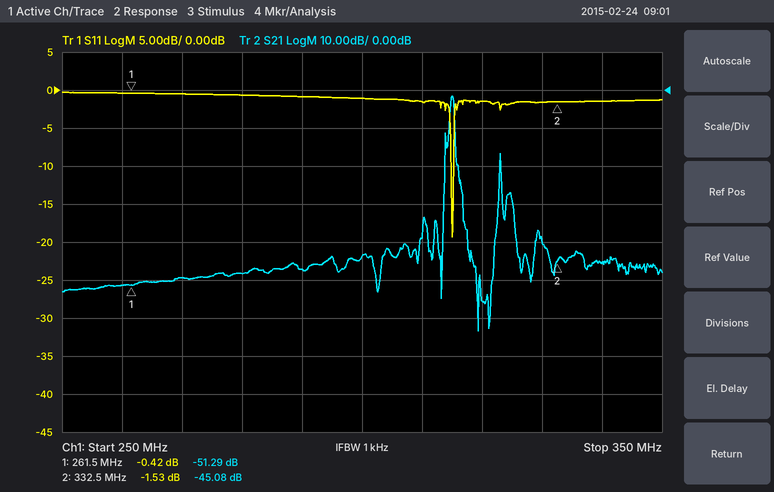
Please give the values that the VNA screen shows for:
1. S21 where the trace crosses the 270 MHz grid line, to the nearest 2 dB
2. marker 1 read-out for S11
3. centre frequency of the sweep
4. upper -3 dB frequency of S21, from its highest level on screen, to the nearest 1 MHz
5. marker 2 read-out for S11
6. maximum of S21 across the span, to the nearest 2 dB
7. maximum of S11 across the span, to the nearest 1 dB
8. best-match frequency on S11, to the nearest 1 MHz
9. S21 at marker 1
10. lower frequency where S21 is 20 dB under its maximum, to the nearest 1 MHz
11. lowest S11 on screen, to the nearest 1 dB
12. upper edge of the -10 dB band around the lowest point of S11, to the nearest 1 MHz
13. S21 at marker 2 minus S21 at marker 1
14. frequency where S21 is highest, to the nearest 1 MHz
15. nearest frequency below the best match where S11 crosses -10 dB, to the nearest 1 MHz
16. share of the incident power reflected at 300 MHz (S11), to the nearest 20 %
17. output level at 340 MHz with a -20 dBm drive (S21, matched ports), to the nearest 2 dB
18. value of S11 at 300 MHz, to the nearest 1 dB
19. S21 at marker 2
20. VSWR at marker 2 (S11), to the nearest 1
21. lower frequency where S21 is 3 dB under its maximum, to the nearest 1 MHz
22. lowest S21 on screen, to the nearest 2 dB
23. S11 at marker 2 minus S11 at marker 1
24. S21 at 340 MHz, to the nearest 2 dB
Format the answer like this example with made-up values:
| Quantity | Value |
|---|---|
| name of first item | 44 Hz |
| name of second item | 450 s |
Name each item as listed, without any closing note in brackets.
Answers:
| Quantity | Value |
|---|---|
| S21 where the trace crosses the 270 MHz grid line, to the nearest 2 dB | -50 dB |
| marker 1 read-out for S11 | -0.42 dB |
| centre frequency of the sweep | 300 MHz |
| upper -3 dB frequency of S21, from its highest level on screen, to the nearest 1 MHz | 315 MHz |
| marker 2 read-out for S11 | -1.53 dB |
| maximum of S21 across the span, to the nearest 2 dB | -2 dB |
| maximum of S11 across the span, to the nearest 1 dB | 0 dB |
| best-match frequency on S11, to the nearest 1 MHz | 315 MHz |
| S21 at marker 1 | -51.29 dB |
| lower frequency where S21 is 20 dB under its maximum, to the nearest 1 MHz | 314 MHz |
| lowest S11 on screen, to the nearest 1 dB | -19 dB |
| upper edge of the -10 dB band around the lowest point of S11, to the nearest 1 MHz | 315 MHz |
| S21 at marker 2 minus S21 at marker 1 | 6.21 dB |
| frequency where S21 is highest, to the nearest 1 MHz | 315 MHz |
| nearest frequency below the best match where S11 crosses -10 dB, to the nearest 1 MHz | 315 MHz |
| share of the incident power reflected at 300 MHz (S11), to the nearest 20 % | 80 % |
| output level at 340 MHz with a -20 dBm drive (S21, matched ports), to the nearest 2 dB | -66 dBm |
| value of S11 at 300 MHz, to the nearest 1 dB | -1 dB |
| S21 at marker 2 | -45.08 dB |
| VSWR at marker 2 (S11), to the nearest 1 | 11 |
| lower frequency where S21 is 3 dB under its maximum, to the nearest 1 MHz | 315 MHz |
| lowest S21 on screen, to the nearest 2 dB | -64 dB |
| S11 at marker 2 minus S11 at marker 1 | -1.11 dB |
| S21 at 340 MHz, to the nearest 2 dB | -46 dB |
